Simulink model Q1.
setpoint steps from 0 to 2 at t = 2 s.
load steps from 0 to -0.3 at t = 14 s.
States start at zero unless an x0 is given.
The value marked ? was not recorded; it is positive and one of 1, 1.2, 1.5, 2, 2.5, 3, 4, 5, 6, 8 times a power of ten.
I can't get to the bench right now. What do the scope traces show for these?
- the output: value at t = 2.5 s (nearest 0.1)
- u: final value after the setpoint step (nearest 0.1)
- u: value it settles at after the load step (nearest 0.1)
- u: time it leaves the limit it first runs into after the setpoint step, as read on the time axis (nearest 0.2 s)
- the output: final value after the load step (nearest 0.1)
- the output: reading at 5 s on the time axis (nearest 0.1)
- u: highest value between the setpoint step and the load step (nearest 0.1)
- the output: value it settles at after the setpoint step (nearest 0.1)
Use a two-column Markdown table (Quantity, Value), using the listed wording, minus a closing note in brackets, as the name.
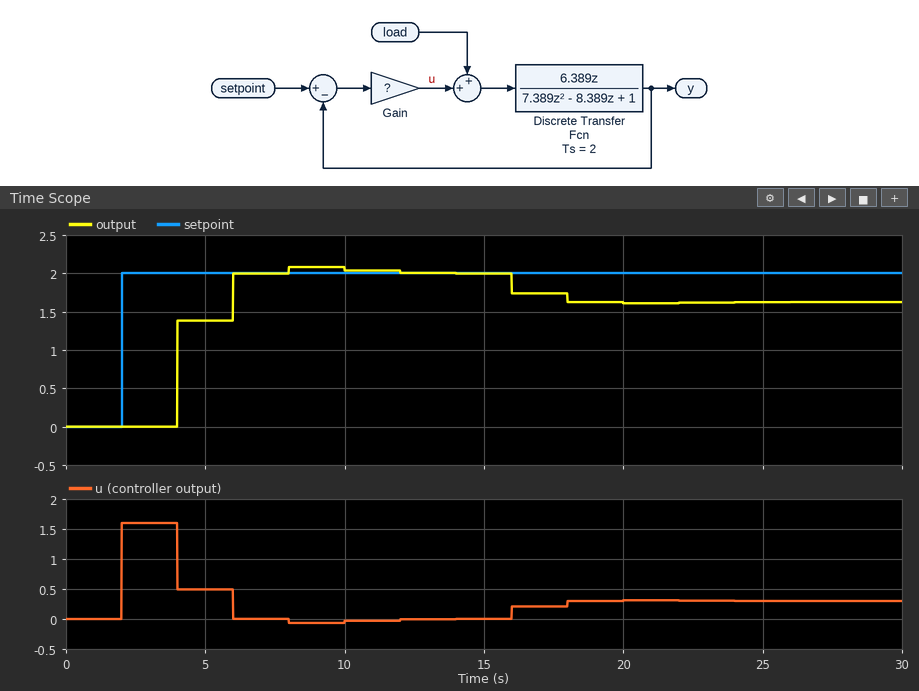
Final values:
| Quantity | Value |
|---|---|
| the output: value at t = 2.5 s | 0.0 |
| u: final value after the setpoint step | 0.0 |
| u: value it settles at after the load step | 0.3 |
| u: time it leaves the limit it first runs into after the setpoint step, as read on the time axis | 4.0 s |
| the output: final value after the load step | 1.6 |
| the output: reading at 5 s on the time axis | 1.4 |
| u: highest value between the setpoint step and the load step | 1.6 |
| the output: value it settles at after the setpoint step | 2.0 |
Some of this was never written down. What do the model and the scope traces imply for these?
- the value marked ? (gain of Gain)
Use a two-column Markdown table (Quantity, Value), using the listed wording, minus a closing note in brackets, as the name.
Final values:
| Quantity | Value |
|---|---|
| the value marked ? | 0.8 |
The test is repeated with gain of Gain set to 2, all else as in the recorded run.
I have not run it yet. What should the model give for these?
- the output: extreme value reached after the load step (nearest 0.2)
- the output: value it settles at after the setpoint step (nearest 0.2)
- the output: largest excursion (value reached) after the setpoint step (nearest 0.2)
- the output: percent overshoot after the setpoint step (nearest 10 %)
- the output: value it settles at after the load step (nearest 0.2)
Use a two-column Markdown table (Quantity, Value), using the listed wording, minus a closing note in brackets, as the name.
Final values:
| Quantity | Value |
|---|---|
| the output: extreme value reached after the load step | 1.8 |
| the output: value it settles at after the setpoint step | 2.0 |
| the output: largest excursion (value reached) after the setpoint step | 3.4 |
| the output: percent overshoot after the setpoint step | 70 % |
| the output: value it settles at after the load step | 1.8 |
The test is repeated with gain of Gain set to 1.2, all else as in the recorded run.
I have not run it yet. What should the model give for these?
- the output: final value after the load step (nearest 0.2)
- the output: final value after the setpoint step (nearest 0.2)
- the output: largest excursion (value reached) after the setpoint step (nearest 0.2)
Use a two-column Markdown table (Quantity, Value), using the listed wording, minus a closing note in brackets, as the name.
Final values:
| Quantity | Value |
|---|---|
| the output: final value after the load step | 1.8 |
| the output: final value after the setpoint step | 2.0 |
| the output: largest excursion (value reached) after the setpoint step | 2.2 |
